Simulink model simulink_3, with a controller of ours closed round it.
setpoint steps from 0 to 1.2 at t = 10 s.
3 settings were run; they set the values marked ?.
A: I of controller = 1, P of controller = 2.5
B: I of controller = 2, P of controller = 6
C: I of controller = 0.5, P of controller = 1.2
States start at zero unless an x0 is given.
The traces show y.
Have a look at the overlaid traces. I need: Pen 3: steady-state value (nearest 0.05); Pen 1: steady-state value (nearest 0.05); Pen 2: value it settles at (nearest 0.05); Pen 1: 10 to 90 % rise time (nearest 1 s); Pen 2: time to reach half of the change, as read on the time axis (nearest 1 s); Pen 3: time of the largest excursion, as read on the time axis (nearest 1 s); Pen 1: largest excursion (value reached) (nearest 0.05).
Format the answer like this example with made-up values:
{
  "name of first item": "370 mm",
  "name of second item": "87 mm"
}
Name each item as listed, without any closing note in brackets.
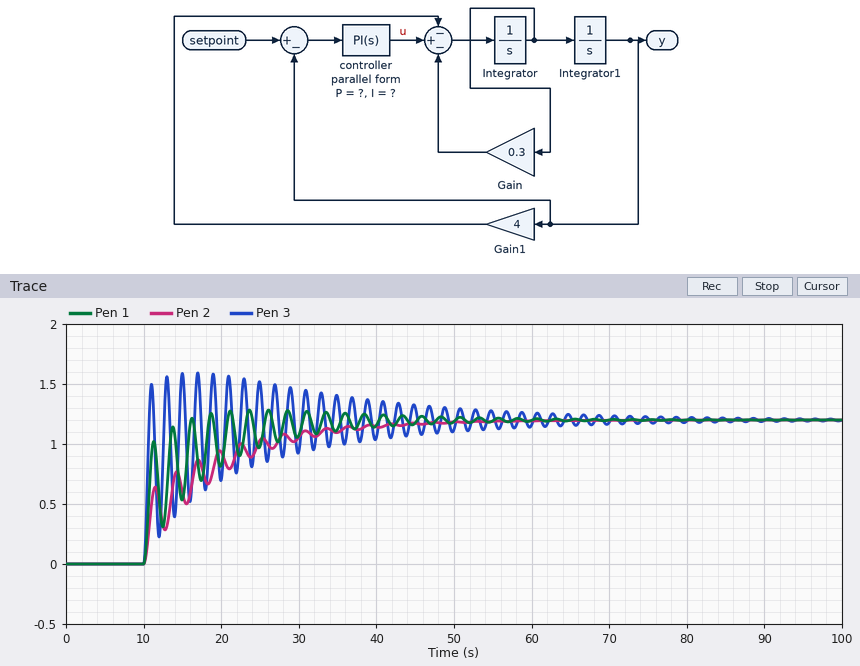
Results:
{
  "Pen 3: steady-state value": "1.20",
  "Pen 1: steady-state value": "1.20",
  "Pen 2: value it settles at": "1.20",
  "Pen 1: 10 to 90 % rise time": "3 s",
  "Pen 2: time to reach half of the change, as read on the time axis": "11 s",
  "Pen 3: time of the largest excursion, as read on the time axis": "17 s",
  "Pen 1: largest excursion (value reached)": "1.30"
}
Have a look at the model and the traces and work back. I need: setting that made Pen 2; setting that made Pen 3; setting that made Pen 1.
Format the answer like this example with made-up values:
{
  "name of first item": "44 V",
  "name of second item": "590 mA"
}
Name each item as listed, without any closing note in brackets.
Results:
{
  "setting that made Pen 2": "C",
  "setting that made Pen 3": "B",
  "setting that made Pen 1": "A"
}
